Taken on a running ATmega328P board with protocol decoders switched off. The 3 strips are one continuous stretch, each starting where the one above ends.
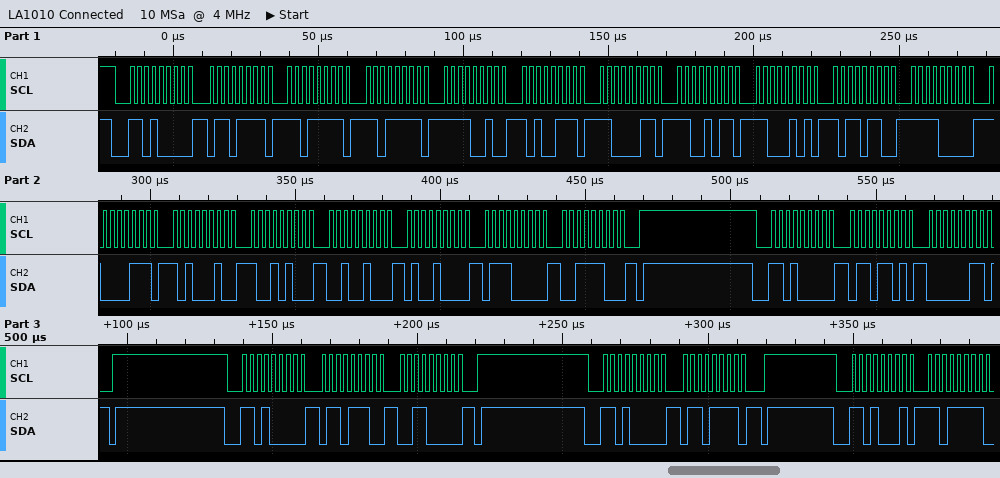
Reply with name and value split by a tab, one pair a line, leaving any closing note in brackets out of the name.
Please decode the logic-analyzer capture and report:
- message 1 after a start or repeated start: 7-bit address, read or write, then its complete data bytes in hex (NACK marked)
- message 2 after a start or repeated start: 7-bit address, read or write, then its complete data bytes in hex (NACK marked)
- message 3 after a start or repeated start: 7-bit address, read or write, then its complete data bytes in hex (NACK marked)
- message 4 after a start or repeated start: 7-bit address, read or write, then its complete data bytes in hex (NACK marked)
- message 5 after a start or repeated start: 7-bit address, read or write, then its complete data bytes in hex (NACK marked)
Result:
message 1 after a start or repeated start: 7-bit address, read or write, then its complete data bytes in hex	0x68 write: 6F DF DF F2 A7 C3 CB C5 B6 F0 87 A2 94 24 48 70 3C
message 2 after a start or repeated start: 7-bit address, read or write, then its complete data bytes in hex	0x68 write: 6D 03
message 3 after a start or repeated start: 7-bit address, read or write, then its complete data bytes in hex	0x68 write: 6E 30
message 4 after a start or repeated start: 7-bit address, read or write, then its complete data bytes in hex	0x68 write: 6F
message 5 after a start or repeated start: 7-bit address, read or write, then its complete data bytes in hex	0x68 read: DF
